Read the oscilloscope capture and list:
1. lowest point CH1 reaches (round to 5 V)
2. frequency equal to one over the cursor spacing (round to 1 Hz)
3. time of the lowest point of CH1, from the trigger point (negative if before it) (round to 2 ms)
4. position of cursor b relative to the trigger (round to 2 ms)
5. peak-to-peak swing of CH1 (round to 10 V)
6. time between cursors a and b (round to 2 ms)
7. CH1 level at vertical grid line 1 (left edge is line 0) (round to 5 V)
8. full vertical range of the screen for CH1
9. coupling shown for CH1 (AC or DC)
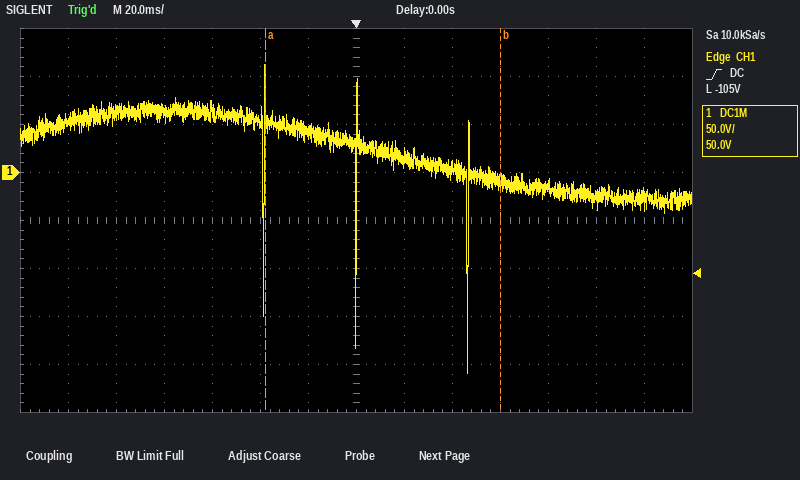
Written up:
-210 V
10 Hz
+46 ms
+60 ms
320 V
98 ms
55 V
400 V
DC
